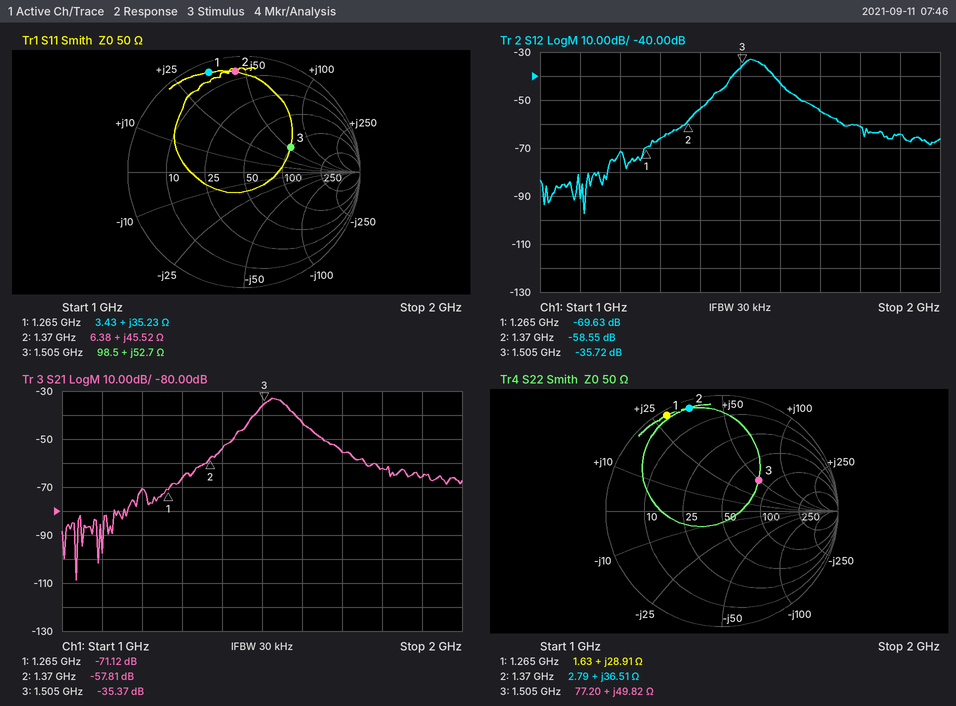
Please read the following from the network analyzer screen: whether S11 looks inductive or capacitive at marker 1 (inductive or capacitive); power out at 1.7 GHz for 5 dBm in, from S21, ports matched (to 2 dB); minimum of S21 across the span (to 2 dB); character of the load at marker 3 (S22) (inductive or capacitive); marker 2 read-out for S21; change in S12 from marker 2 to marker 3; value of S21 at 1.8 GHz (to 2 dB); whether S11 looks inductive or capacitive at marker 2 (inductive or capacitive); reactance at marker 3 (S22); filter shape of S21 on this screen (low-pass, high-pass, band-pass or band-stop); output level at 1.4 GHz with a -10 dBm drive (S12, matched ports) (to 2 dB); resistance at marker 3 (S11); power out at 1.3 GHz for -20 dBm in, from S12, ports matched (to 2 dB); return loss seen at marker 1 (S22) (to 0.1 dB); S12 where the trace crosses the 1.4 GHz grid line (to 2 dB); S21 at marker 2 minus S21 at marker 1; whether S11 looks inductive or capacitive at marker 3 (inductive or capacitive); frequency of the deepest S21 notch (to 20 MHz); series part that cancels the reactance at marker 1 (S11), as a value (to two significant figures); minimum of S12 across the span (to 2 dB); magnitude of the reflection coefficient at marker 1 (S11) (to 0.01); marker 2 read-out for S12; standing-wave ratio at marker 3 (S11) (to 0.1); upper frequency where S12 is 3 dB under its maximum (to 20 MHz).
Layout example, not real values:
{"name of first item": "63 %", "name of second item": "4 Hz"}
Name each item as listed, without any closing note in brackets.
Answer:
{"whether S11 looks inductive or capacitive at marker 1": "inductive", "power out at 1.7 GHz for 5 dBm in, from S21, ports matched": "-50 dBm", "minimum of S21 across the span": "-108 dB", "character of the load at marker 3 (S22)": "inductive", "marker 2 read-out for S21": "-57.81 dB", "change in S12 from marker 2 to marker 3": "22.83 dB", "value of S21 at 1.8 GHz": "-62 dB", "whether S11 looks inductive or capacitive at marker 2": "inductive", "reactance at marker 3": "+49.82 Ω", "filter shape of S21 on this screen": "band-pass", "output level at 1.4 GHz with a -10 dBm drive (S12, matched ports)": "-64 dBm", "resistance at marker 3": "98.5 Ω", "power out at 1.3 GHz for -20 dBm in, from S12, ports matched": "-86 dBm", "return loss seen at marker 1 (S22)": "0.4 dB", "S12 where the trace crosses the 1.4 GHz grid line": "-54 dB", "S21 at marker 2 minus S21 at marker 1": "13.31 dB", "whether S11 looks inductive or capacitive at marker 3": "inductive", "frequency of the deepest S21 notch": "1.04 GHz", "series part that cancels the reactance at marker 1 (S11), as a value": "3.6 pF", "minimum of S12 across the span": "-98 dB", "magnitude of the reflection coefficient at marker 1 (S11)": "0.91", "marker 2 read-out for S12": "-58.55 dB", "standing-wave ratio at marker 3 (S11)": "2.7", "upper frequency where S12 is 3 dB under its maximum": "1.56 GHz"}
